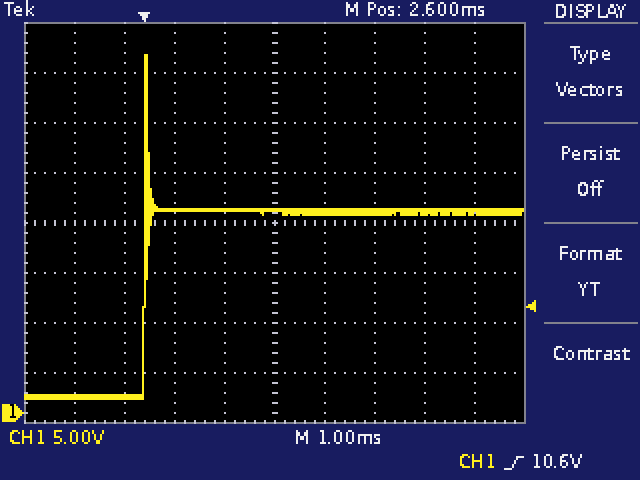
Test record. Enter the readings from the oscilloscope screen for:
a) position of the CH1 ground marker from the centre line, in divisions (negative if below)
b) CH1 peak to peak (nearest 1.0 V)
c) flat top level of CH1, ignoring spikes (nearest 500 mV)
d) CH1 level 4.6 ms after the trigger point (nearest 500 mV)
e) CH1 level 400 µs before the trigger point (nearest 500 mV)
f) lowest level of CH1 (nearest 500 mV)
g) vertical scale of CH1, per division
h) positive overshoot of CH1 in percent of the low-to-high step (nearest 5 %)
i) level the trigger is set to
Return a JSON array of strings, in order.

["-3.8 div", "34.0 V", "20.0 V", "20.0 V", "1.5 V", "1.5 V", "5 V", "85 %", "10.6 V"]
